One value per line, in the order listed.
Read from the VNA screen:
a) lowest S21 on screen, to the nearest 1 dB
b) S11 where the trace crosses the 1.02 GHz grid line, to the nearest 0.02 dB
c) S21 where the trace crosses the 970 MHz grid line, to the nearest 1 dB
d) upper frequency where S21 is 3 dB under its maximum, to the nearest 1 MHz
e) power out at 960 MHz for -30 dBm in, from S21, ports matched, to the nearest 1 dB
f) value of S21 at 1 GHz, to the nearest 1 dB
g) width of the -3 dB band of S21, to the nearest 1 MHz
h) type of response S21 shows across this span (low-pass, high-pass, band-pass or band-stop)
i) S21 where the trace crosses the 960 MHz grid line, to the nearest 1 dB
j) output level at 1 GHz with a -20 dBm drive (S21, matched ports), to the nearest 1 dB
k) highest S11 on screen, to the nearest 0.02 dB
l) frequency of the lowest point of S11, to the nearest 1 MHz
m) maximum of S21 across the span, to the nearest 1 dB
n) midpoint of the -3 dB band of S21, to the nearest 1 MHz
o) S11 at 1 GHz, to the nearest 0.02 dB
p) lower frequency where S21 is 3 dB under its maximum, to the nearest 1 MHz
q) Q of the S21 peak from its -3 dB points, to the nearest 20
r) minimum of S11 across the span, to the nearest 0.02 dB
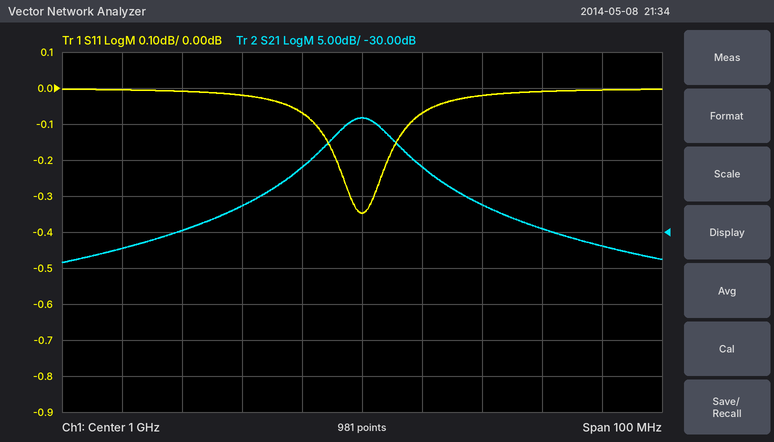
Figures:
-34 dB
-0.02 dB
-30 dB
1.005 GHz
-62 dBm
-14 dB
10 MHz
band-pass
-32 dB
-34 dBm
0.00 dB
1.000 GHz
-14 dB
1.000 GHz
-0.34 dB
995 MHz
100
-0.34 dB
